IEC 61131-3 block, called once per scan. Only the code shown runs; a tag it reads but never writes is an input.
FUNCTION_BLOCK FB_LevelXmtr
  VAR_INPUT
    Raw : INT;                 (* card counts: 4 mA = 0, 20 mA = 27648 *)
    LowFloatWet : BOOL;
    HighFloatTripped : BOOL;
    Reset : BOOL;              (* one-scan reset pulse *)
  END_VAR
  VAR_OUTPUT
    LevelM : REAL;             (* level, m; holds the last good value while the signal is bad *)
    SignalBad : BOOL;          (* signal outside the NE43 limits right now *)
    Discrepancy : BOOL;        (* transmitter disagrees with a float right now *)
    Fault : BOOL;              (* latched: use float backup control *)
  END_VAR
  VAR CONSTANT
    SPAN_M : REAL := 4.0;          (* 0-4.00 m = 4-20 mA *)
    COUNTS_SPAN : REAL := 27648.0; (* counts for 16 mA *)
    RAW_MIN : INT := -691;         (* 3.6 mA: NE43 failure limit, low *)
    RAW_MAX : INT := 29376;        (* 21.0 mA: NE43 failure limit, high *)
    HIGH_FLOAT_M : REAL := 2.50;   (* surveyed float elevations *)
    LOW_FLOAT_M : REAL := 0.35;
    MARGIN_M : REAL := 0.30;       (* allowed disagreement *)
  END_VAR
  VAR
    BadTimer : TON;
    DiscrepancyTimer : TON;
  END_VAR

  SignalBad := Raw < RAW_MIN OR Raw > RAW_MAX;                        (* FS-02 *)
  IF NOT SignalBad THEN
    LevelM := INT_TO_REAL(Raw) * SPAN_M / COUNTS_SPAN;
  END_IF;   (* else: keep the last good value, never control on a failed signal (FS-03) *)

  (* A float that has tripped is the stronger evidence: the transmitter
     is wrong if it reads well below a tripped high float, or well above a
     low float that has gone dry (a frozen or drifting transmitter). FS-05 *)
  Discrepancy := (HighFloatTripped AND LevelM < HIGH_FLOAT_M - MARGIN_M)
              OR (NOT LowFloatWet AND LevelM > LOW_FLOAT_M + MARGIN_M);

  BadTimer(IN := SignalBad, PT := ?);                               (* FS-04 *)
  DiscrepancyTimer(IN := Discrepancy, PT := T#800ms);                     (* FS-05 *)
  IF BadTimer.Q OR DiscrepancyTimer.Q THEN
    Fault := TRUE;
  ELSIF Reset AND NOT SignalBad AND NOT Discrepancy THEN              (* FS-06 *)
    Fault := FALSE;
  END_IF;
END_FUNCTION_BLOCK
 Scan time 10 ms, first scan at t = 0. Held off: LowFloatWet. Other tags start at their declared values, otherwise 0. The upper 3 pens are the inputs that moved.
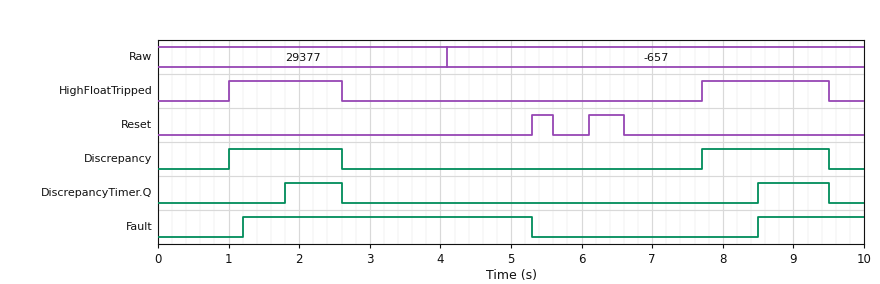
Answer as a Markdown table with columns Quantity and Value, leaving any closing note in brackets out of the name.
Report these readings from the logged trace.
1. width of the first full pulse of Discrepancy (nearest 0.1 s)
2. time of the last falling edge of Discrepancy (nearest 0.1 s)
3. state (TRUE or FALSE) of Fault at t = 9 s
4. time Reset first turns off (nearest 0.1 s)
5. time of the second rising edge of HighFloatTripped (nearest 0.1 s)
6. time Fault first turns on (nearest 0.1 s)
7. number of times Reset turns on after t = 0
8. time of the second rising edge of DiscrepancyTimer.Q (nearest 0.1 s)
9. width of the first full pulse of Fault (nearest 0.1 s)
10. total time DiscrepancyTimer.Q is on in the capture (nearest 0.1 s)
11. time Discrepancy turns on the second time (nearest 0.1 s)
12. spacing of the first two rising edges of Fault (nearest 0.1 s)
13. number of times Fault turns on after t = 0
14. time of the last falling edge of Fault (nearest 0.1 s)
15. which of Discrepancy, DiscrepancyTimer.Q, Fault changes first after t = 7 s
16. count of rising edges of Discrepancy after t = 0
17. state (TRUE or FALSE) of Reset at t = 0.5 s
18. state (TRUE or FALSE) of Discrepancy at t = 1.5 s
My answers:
| Quantity | Value |
|---|---|
| width of the first full pulse of Discrepancy | 1.6 s |
| time of the last falling edge of Discrepancy | 9.5 s |
| state (TRUE or FALSE) of Fault at t = 9 s | TRUE |
| time Reset first turns off | 5.6 s |
| time of the second rising edge of HighFloatTripped | 7.7 s |
| time Fault first turns on | 1.2 s |
| number of times Reset turns on after t = 0 | 2 |
| time of the second rising edge of DiscrepancyTimer.Q | 8.5 s |
| width of the first full pulse of Fault | 4.1 s |
| total time DiscrepancyTimer.Q is on in the capture | 1.8 s |
| time Discrepancy turns on the second time | 7.7 s |
| spacing of the first two rising edges of Fault | 7.3 s |
| number of times Fault turns on after t = 0 | 2 |
| time of the last falling edge of Fault | 5.3 s |
| which of Discrepancy, DiscrepancyTimer.Q, Fault changes first after t = 7 s | Discrepancy |
| count of rising edges of Discrepancy after t = 0 | 2 |
| state (TRUE or FALSE) of Reset at t = 0.5 s | FALSE |
| state (TRUE or FALSE) of Discrepancy at t = 1.5 s | TRUE |
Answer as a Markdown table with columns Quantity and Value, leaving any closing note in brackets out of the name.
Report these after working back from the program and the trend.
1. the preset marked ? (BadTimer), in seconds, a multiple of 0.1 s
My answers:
| Quantity | Value |
|---|---|
| the preset marked ? (BadTimer), in seconds, a multiple of 0.1 s | 1.2 s |
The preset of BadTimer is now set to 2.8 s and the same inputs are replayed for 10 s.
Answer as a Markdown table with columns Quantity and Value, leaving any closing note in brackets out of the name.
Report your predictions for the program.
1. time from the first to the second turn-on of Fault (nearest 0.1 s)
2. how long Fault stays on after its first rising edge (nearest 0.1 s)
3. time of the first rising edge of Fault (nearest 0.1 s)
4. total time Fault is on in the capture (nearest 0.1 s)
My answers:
| Quantity | Value |
|---|---|
| time from the first to the second turn-on of Fault | 6.7 s |
| how long Fault stays on after its first rising edge | 3.5 s |
| time of the first rising edge of Fault | 1.8 s |
| total time Fault is on in the capture | 5.0 s |
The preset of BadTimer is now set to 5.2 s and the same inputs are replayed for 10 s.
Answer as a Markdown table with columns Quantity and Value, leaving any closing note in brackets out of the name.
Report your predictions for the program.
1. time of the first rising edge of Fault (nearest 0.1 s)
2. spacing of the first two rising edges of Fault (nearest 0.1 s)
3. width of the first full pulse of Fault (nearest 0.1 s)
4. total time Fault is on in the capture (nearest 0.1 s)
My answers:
| Quantity | Value |
|---|---|
| time of the first rising edge of Fault | 1.8 s |
| spacing of the first two rising edges of Fault | 6.7 s |
| width of the first full pulse of Fault | 3.5 s |
| total time Fault is on in the capture | 5.0 s |
